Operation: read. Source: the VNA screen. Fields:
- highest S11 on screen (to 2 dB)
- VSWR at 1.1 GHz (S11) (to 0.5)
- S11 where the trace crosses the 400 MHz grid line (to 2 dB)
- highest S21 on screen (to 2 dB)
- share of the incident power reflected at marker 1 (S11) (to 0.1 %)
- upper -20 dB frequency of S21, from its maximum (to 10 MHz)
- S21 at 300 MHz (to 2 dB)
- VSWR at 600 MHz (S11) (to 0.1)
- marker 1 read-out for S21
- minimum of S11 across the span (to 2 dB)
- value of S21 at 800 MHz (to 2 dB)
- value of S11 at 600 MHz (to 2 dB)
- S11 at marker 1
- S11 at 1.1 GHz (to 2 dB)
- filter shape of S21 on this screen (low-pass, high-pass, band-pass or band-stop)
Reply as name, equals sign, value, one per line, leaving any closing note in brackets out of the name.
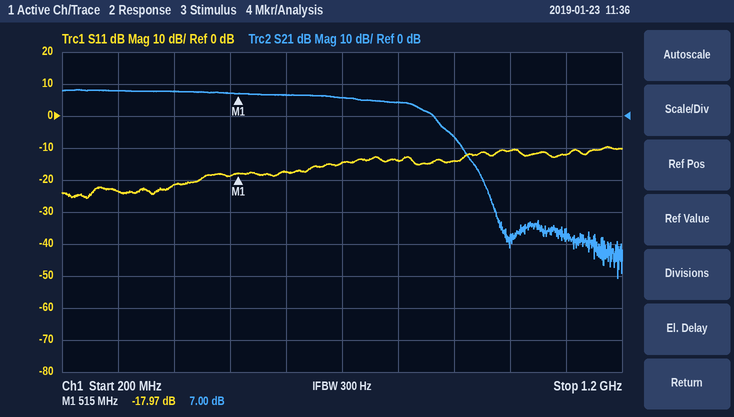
highest S11 on screen = -10 dB
VSWR at 1.1 GHz (S11) = 1.5
S11 where the trace crosses the 400 MHz grid line = -22 dB
highest S21 on screen = 8 dB
share of the incident power reflected at marker 1 (S11) = 1.6 %
upper -20 dB frequency of S21, from its maximum = 920 MHz
S21 at 300 MHz = 8 dB
VSWR at 600 MHz (S11) = 1.3
marker 1 read-out for S21 = 7.00 dB
minimum of S11 across the span = -26 dB
value of S21 at 800 MHz = 4 dB
value of S11 at 600 MHz = -18 dB
S11 at marker 1 = -17.97 dB
S11 at 1.1 GHz = -12 dB
filter shape of S21 on this screen = low-pass
